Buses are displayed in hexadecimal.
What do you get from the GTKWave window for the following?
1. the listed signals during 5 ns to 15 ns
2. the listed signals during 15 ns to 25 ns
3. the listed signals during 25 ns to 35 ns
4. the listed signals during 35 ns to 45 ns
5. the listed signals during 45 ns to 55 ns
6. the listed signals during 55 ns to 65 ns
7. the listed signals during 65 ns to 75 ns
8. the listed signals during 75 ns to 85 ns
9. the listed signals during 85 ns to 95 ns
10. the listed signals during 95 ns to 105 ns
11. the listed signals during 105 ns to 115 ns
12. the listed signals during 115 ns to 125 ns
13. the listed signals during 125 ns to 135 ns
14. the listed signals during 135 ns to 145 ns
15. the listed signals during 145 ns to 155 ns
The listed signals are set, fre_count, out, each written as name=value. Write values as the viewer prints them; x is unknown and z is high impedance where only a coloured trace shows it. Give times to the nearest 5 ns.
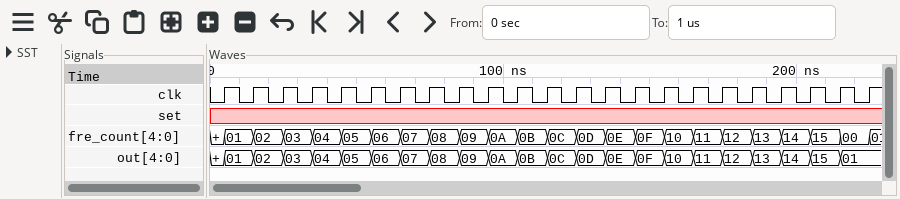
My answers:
set=x, fre_count=01, out=01
set=x, fre_count=02, out=02
set=x, fre_count=03, out=03
set=x, fre_count=04, out=04
set=x, fre_count=05, out=05
set=x, fre_count=06, out=06
set=x, fre_count=07, out=07
set=x, fre_count=08, out=08
set=x, fre_count=09, out=09
set=x, fre_count=0A, out=0A
set=x, fre_count=0B, out=0B
set=x, fre_count=0C, out=0C
set=x, fre_count=0D, out=0D
set=x, fre_count=0E, out=0E
set=x, fre_count=0F, out=0F
